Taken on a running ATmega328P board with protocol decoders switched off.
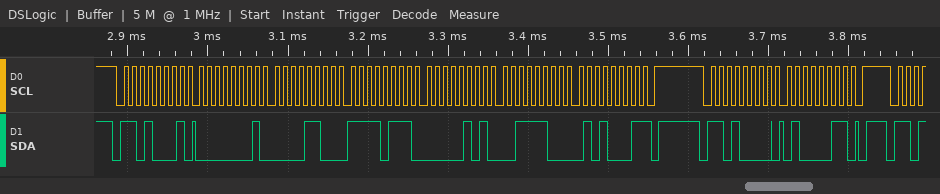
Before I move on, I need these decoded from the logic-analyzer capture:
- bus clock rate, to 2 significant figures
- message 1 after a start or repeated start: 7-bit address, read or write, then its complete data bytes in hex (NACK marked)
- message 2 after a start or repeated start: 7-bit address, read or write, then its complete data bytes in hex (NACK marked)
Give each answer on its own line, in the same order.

100 kHz
0x68 read: 01 0C F7 05 3C 51 NACK
0x68 write: 43
